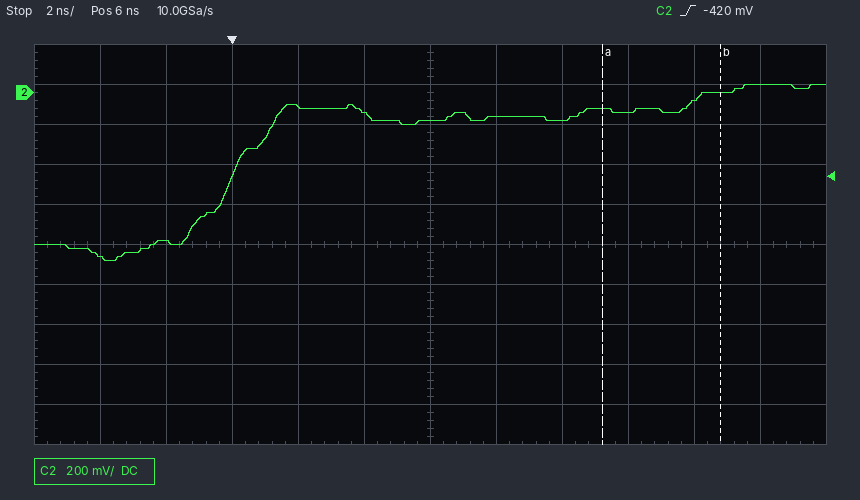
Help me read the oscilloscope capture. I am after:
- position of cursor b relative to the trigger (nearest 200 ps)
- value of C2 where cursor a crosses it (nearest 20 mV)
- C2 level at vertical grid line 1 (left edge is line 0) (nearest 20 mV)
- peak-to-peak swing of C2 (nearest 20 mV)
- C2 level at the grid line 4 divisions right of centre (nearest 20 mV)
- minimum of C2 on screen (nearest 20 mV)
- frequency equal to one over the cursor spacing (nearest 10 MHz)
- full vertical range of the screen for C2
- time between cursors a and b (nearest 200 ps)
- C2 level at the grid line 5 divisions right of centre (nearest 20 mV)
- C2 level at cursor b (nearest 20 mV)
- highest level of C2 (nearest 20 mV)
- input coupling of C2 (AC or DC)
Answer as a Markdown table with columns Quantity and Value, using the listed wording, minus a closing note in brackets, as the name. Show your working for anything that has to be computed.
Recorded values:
| Quantity | Value |
|---|---|
| position of cursor b relative to the trigger | +14.8 ns |
| value of C2 where cursor a crosses it | -80 mV |
| C2 level at vertical grid line 1 (left edge is line 0) | -820 mV |
| peak-to-peak swing of C2 | 40 mV − (-840 mV) = 880 mV |
| C2 level at the grid line 4 divisions right of centre | -40 mV |
| minimum of C2 on screen | -840 mV |
| frequency equal to one over the cursor spacing | 1 / 3.6 ns ≈ 280 MHz |
| full vertical range of the screen for C2 | 2 V |
| time between cursors a and b | 3.6 ns |
| C2 level at the grid line 5 divisions right of centre | 40 mV |
| C2 level at cursor b | 0 mV |
| highest level of C2 | 40 mV |
| input coupling of C2 | DC |
